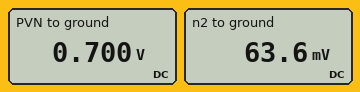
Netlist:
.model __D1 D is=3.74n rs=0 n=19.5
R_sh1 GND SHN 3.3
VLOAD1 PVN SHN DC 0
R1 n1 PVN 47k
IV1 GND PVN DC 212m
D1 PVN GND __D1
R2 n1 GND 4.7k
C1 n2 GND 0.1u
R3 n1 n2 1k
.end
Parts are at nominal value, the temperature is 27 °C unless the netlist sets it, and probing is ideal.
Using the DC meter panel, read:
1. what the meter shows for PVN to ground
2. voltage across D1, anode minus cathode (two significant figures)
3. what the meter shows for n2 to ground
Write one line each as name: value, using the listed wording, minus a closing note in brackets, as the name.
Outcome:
what the meter shows for PVN to ground: 0.700 V
voltage across D1, anode minus cathode: 700 mV
what the meter shows for n2 to ground: 63.6 mV
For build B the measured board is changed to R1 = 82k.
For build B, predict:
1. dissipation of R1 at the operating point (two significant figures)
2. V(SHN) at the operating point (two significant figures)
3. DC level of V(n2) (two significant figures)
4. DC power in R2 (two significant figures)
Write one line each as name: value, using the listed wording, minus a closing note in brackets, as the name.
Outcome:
dissipation of R1 at the operating point: 5.3 µW
V(SHN) at the operating point: 700 mV
DC level of V(n2): 38 mV
DC power in R2: 310 nW
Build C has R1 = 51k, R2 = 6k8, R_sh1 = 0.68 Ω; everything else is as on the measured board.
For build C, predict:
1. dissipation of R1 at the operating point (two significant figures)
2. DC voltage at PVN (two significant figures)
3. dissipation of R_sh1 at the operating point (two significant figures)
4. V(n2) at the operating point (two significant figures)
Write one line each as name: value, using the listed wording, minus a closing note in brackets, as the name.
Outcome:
dissipation of R1 at the operating point: 320 nW
DC voltage at PVN: 140 mV
dissipation of R_sh1 at the operating point: 31 mW
V(n2) at the operating point: 17 mV
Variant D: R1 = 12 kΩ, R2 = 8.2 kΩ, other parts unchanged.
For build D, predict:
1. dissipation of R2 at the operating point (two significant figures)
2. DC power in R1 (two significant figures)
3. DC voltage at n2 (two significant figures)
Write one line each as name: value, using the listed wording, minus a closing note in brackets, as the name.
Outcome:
dissipation of R2 at the operating point: 9.8 µW
DC power in R1: 14 µW
DC voltage at n2: 280 mV
